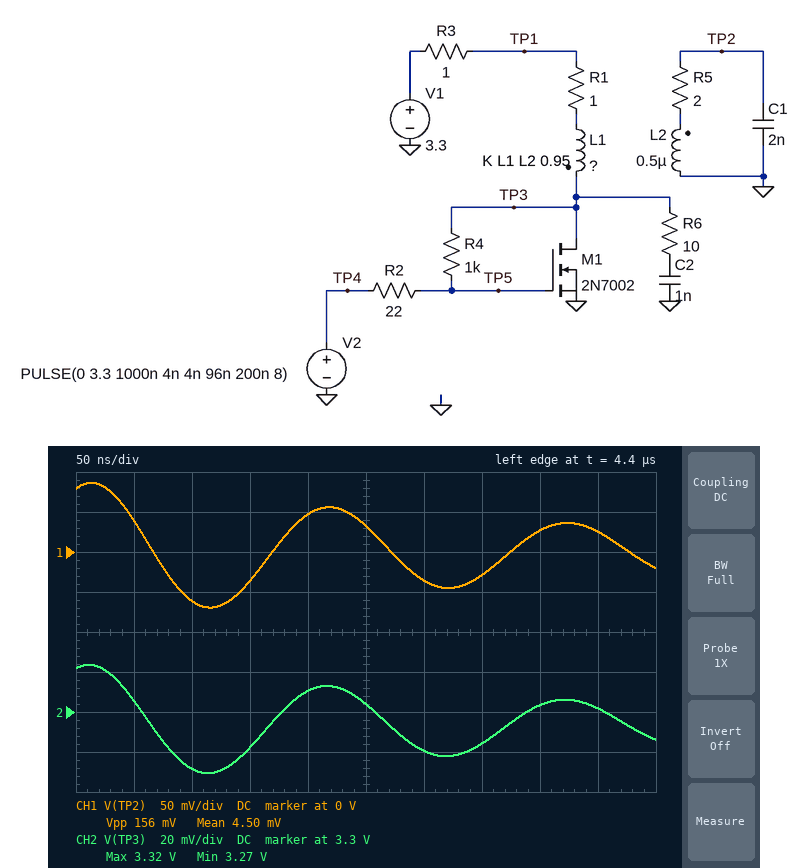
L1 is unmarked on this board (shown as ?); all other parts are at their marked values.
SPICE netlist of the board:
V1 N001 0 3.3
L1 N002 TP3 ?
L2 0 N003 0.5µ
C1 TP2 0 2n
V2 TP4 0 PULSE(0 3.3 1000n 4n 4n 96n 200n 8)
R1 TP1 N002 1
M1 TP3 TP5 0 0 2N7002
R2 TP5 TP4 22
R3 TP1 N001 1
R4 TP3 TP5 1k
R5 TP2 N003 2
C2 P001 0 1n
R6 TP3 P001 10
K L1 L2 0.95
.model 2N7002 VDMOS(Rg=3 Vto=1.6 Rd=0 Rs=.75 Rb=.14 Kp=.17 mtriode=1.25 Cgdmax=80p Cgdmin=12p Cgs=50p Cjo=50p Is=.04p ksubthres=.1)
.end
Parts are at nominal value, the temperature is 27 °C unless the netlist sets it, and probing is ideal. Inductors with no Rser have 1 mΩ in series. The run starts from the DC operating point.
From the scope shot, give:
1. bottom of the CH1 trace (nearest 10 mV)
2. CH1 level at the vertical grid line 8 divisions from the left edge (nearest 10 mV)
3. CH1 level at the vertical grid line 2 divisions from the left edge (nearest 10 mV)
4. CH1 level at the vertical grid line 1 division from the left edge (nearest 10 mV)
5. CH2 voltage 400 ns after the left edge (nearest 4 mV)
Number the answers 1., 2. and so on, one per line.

1. -70 mV
2. 30 mV
3. -60 mV
4. 40 mV
5. 3.304 V
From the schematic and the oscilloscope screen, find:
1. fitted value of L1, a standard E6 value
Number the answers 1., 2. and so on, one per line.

1. 68 nH
